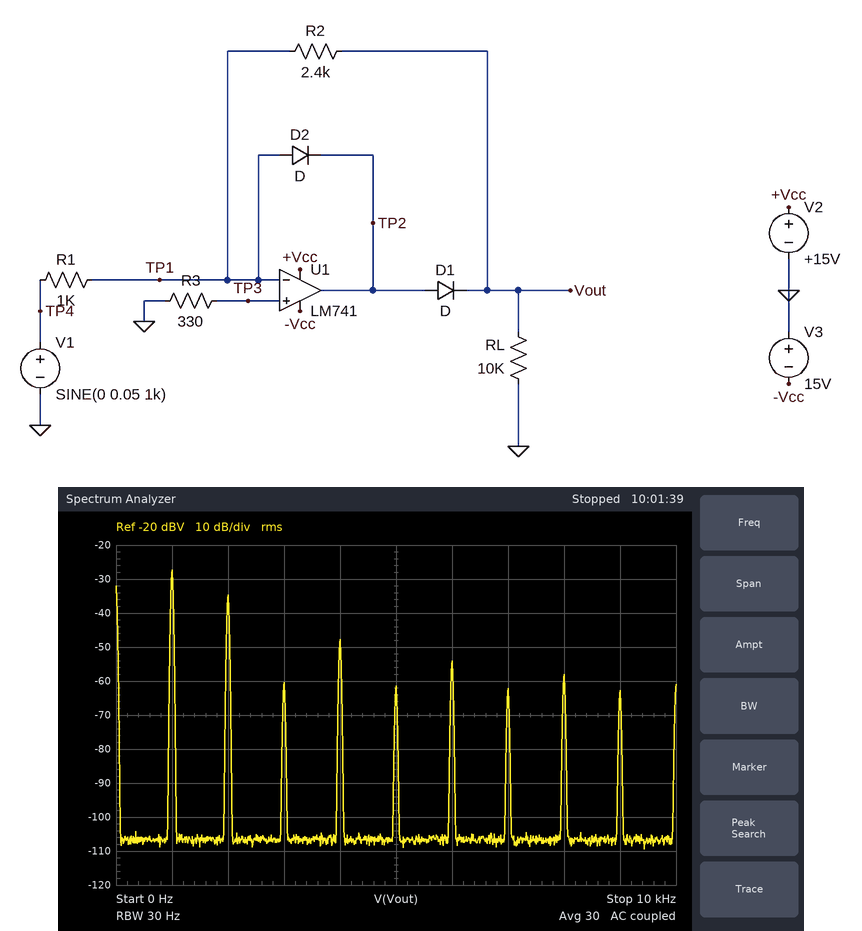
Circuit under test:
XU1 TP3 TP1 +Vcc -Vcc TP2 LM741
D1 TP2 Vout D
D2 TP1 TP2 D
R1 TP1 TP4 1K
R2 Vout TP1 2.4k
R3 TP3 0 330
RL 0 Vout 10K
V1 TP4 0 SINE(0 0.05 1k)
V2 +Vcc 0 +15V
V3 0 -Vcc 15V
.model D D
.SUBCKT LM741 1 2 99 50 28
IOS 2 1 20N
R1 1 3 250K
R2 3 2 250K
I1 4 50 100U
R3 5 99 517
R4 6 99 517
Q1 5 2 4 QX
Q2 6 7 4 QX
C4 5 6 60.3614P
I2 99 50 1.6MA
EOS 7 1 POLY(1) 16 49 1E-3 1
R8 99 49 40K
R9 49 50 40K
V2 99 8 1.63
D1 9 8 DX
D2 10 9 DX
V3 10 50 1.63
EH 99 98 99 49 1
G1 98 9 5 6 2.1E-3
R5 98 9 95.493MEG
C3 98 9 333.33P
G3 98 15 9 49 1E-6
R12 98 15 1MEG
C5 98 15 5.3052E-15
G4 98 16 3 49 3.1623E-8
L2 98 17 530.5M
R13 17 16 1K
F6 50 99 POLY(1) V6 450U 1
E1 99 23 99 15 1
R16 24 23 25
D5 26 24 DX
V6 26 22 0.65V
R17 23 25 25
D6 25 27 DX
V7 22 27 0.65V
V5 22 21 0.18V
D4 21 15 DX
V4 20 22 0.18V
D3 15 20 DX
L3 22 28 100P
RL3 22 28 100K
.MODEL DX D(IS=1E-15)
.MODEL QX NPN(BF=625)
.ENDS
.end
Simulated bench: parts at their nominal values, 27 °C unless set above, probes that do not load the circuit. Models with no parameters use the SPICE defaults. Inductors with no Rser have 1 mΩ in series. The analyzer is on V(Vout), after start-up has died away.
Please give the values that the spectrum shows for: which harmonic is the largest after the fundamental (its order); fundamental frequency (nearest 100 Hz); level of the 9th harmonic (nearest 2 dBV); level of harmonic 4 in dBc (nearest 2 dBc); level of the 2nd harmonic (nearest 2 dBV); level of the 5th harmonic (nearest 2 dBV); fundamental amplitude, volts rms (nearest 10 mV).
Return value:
2
1.0 kHz
-62 dBV
-20 dBc
-34 dBV
-62 dBV
40 mV
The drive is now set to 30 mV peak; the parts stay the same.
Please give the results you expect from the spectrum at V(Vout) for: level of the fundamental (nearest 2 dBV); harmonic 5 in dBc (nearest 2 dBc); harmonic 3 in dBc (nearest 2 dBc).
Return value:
-32 dBV
-30 dBc
-30 dBc
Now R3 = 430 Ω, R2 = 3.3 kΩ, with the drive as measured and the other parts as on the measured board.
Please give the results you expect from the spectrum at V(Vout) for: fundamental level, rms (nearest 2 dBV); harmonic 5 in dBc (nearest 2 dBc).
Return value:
-24 dBV
-36 dBc
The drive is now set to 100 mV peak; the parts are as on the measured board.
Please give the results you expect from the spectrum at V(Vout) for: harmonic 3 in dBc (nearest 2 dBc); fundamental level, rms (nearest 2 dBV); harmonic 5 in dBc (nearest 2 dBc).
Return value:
-38 dBc
-22 dBV
-40 dBc
